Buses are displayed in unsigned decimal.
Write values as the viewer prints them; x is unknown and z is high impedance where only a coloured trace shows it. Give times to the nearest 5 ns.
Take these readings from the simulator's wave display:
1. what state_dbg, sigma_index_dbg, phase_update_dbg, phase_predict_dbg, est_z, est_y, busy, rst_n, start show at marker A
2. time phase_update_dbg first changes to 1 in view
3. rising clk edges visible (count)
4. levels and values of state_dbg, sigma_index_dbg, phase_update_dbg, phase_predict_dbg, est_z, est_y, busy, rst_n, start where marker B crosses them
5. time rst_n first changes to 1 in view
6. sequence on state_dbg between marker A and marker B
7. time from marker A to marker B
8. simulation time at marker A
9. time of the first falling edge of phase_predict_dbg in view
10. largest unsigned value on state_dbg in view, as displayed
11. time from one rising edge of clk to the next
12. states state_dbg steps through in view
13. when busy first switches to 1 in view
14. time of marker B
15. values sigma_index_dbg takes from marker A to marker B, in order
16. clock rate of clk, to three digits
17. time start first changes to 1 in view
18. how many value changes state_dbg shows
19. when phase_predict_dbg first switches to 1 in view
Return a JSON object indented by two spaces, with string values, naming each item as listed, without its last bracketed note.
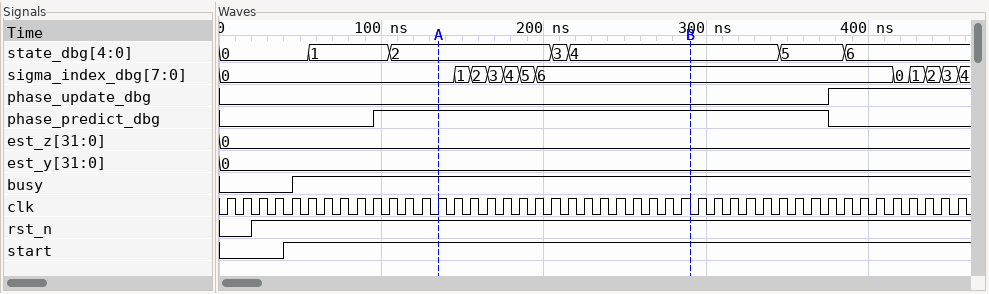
{
  "what state_dbg, sigma_index_dbg, phase_update_dbg, phase_predict_dbg, est_z, est_y, busy, rst_n, start show at marker A": "state_dbg=2, sigma_index_dbg=0, phase_update_dbg=0, phase_predict_dbg=1, est_z=0, est_y=0, busy=1, rst_n=1, start=1",
  "time phase_update_dbg first changes to 1 in view": "375 ns",
  "rising clk edges visible": "46",
  "levels and values of state_dbg, sigma_index_dbg, phase_update_dbg, phase_predict_dbg, est_z, est_y, busy, rst_n, start where marker B crosses them": "state_dbg=4, sigma_index_dbg=6, phase_update_dbg=0, phase_predict_dbg=1, est_z=0, est_y=0, busy=1, rst_n=1, start=1",
  "time rst_n first changes to 1 in view": "20 ns",
  "sequence on state_dbg between marker A and marker B": "2, 3, 4",
  "time from marker A to marker B": "155 ns",
  "simulation time at marker A": "135 ns",
  "time of the first falling edge of phase_predict_dbg in view": "375 ns",
  "largest unsigned value on state_dbg in view, as displayed": "6",
  "time from one rising edge of clk to the next": "10 ns",
  "states state_dbg steps through in view": "0, 1, 2, 3, 4, 5, 6",
  "when busy first switches to 1 in view": "45 ns",
  "time of marker B": "290 ns",
  "values sigma_index_dbg takes from marker A to marker B, in order": "0, 1, 2, 3, 4, 5, 6",
  "clock rate of clk, to three digits": "100 MHz",
  "time start first changes to 1 in view": "40 ns",
  "how many value changes state_dbg shows": "6",
  "when phase_predict_dbg first switches to 1 in view": "95 ns"
}
